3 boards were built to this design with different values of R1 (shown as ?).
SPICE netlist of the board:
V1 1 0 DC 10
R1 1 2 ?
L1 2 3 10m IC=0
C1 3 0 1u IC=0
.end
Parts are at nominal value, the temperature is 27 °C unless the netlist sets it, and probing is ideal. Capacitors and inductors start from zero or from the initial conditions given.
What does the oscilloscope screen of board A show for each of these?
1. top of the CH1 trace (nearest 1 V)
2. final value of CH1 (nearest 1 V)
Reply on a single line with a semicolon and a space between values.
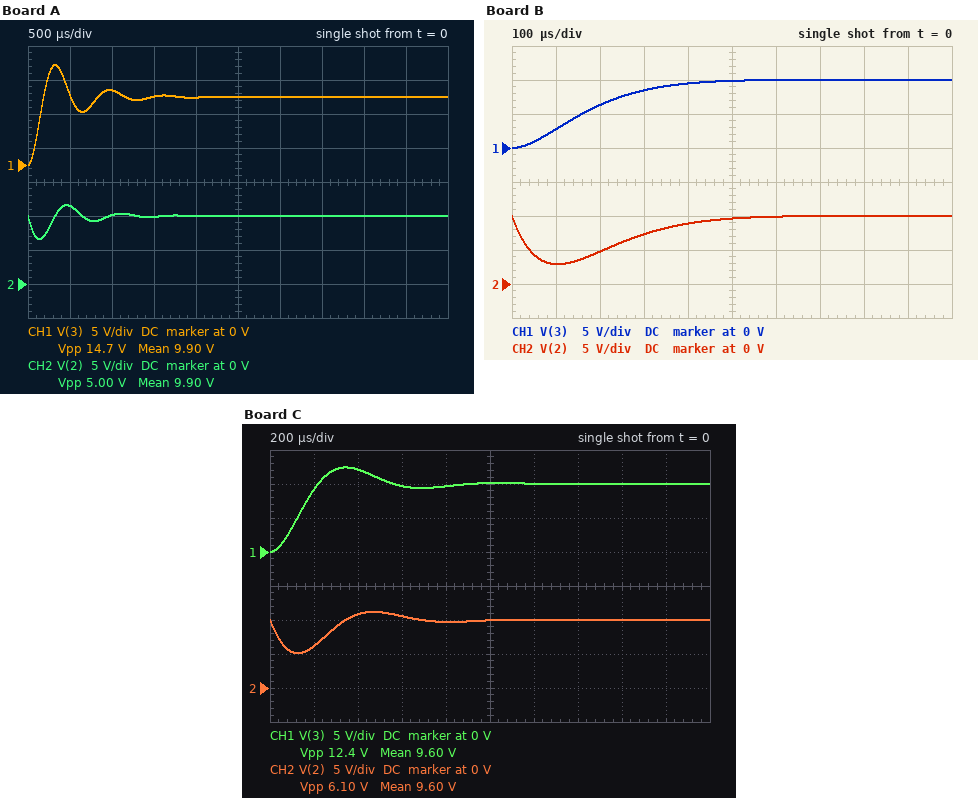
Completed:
15 V; 10 V
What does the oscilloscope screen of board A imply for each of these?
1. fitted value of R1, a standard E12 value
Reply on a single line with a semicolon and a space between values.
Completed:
47 Ω
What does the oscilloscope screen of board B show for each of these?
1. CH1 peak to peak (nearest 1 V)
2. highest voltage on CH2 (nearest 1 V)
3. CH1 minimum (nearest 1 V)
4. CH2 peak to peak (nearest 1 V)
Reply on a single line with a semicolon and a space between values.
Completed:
10 V; 10 V; 0 V; 7 V
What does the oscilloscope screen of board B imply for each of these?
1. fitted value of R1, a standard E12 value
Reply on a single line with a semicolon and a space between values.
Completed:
180 Ω
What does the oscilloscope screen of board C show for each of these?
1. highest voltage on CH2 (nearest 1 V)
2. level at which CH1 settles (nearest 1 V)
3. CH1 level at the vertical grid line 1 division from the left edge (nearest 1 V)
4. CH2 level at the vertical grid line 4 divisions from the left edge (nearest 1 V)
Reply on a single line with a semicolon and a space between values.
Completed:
11 V; 10 V; 9 V; 10 V
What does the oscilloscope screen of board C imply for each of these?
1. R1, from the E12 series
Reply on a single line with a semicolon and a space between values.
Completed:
82 Ω
